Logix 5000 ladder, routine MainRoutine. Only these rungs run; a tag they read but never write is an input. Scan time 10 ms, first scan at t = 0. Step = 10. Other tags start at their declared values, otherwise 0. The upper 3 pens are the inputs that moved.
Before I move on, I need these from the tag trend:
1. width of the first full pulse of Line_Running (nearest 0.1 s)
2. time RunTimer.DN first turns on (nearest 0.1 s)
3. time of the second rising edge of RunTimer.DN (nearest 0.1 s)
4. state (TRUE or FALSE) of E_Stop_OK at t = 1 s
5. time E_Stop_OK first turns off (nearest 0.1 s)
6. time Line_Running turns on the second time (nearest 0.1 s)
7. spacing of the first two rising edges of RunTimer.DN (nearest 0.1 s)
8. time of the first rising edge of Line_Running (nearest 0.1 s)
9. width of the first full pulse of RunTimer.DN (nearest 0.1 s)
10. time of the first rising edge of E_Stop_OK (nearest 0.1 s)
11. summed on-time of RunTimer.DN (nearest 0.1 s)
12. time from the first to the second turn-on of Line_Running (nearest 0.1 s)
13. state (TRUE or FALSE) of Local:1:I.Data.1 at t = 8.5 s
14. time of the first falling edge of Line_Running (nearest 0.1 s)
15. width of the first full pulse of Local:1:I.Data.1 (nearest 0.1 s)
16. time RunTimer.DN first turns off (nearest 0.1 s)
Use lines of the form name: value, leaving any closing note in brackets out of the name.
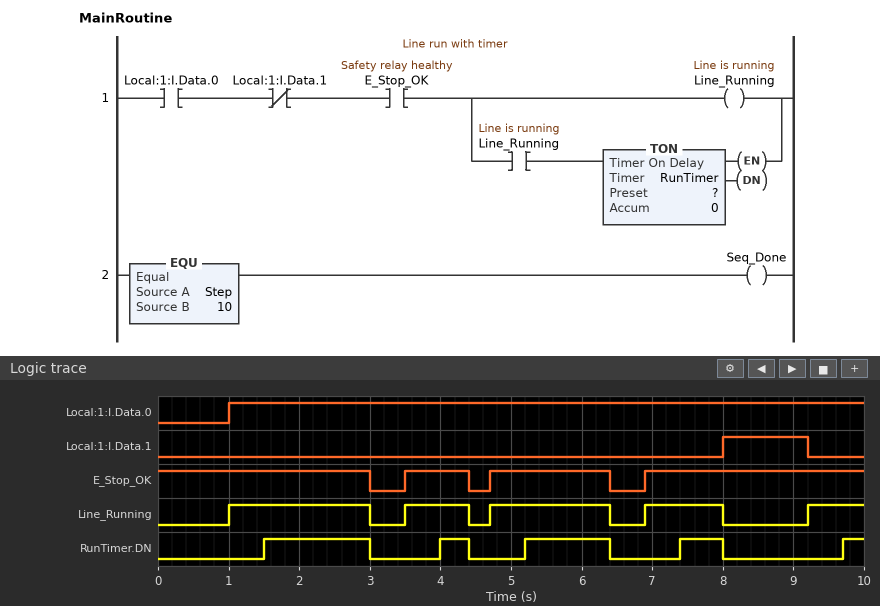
width of the first full pulse of Line_Running: 2.0 s
time RunTimer.DN first turns on: 1.5 s
time of the second rising edge of RunTimer.DN: 4.0 s
state (TRUE or FALSE) of E_Stop_OK at t = 1 s: TRUE
time E_Stop_OK first turns off: 3.0 s
time Line_Running turns on the second time: 3.5 s
spacing of the first two rising edges of RunTimer.DN: 2.5 s
time of the first rising edge of Line_Running: 1.0 s
width of the first full pulse of RunTimer.DN: 1.5 s
time of the first rising edge of E_Stop_OK: 3.5 s
summed on-time of RunTimer.DN: 4.0 s
time from the first to the second turn-on of Line_Running: 2.5 s
state (TRUE or FALSE) of Local:1:I.Data.1 at t = 8.5 s: TRUE
time of the first falling edge of Line_Running: 3.0 s
width of the first full pulse of Local:1:I.Data.1: 1.2 s
time RunTimer.DN first turns off: 3.0 s
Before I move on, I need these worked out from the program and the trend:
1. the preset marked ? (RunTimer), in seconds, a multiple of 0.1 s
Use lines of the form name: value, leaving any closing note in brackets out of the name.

the preset marked ? (RunTimer), in seconds, a multiple of 0.1 s: 0.5 s
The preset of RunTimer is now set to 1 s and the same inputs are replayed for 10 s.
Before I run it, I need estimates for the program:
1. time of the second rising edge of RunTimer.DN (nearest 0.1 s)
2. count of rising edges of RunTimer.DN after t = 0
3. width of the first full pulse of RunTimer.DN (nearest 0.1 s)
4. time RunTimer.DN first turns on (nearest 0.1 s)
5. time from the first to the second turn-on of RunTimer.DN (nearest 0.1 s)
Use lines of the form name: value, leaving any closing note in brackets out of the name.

time of the second rising edge of RunTimer.DN: 5.7 s
count of rising edges of RunTimer.DN after t = 0: 3
width of the first full pulse of RunTimer.DN: 1.0 s
time RunTimer.DN first turns on: 2.0 s
time from the first to the second turn-on of RunTimer.DN: 3.7 s
